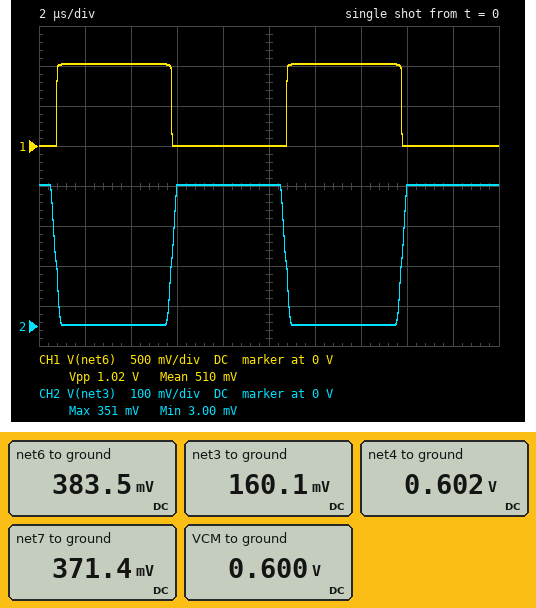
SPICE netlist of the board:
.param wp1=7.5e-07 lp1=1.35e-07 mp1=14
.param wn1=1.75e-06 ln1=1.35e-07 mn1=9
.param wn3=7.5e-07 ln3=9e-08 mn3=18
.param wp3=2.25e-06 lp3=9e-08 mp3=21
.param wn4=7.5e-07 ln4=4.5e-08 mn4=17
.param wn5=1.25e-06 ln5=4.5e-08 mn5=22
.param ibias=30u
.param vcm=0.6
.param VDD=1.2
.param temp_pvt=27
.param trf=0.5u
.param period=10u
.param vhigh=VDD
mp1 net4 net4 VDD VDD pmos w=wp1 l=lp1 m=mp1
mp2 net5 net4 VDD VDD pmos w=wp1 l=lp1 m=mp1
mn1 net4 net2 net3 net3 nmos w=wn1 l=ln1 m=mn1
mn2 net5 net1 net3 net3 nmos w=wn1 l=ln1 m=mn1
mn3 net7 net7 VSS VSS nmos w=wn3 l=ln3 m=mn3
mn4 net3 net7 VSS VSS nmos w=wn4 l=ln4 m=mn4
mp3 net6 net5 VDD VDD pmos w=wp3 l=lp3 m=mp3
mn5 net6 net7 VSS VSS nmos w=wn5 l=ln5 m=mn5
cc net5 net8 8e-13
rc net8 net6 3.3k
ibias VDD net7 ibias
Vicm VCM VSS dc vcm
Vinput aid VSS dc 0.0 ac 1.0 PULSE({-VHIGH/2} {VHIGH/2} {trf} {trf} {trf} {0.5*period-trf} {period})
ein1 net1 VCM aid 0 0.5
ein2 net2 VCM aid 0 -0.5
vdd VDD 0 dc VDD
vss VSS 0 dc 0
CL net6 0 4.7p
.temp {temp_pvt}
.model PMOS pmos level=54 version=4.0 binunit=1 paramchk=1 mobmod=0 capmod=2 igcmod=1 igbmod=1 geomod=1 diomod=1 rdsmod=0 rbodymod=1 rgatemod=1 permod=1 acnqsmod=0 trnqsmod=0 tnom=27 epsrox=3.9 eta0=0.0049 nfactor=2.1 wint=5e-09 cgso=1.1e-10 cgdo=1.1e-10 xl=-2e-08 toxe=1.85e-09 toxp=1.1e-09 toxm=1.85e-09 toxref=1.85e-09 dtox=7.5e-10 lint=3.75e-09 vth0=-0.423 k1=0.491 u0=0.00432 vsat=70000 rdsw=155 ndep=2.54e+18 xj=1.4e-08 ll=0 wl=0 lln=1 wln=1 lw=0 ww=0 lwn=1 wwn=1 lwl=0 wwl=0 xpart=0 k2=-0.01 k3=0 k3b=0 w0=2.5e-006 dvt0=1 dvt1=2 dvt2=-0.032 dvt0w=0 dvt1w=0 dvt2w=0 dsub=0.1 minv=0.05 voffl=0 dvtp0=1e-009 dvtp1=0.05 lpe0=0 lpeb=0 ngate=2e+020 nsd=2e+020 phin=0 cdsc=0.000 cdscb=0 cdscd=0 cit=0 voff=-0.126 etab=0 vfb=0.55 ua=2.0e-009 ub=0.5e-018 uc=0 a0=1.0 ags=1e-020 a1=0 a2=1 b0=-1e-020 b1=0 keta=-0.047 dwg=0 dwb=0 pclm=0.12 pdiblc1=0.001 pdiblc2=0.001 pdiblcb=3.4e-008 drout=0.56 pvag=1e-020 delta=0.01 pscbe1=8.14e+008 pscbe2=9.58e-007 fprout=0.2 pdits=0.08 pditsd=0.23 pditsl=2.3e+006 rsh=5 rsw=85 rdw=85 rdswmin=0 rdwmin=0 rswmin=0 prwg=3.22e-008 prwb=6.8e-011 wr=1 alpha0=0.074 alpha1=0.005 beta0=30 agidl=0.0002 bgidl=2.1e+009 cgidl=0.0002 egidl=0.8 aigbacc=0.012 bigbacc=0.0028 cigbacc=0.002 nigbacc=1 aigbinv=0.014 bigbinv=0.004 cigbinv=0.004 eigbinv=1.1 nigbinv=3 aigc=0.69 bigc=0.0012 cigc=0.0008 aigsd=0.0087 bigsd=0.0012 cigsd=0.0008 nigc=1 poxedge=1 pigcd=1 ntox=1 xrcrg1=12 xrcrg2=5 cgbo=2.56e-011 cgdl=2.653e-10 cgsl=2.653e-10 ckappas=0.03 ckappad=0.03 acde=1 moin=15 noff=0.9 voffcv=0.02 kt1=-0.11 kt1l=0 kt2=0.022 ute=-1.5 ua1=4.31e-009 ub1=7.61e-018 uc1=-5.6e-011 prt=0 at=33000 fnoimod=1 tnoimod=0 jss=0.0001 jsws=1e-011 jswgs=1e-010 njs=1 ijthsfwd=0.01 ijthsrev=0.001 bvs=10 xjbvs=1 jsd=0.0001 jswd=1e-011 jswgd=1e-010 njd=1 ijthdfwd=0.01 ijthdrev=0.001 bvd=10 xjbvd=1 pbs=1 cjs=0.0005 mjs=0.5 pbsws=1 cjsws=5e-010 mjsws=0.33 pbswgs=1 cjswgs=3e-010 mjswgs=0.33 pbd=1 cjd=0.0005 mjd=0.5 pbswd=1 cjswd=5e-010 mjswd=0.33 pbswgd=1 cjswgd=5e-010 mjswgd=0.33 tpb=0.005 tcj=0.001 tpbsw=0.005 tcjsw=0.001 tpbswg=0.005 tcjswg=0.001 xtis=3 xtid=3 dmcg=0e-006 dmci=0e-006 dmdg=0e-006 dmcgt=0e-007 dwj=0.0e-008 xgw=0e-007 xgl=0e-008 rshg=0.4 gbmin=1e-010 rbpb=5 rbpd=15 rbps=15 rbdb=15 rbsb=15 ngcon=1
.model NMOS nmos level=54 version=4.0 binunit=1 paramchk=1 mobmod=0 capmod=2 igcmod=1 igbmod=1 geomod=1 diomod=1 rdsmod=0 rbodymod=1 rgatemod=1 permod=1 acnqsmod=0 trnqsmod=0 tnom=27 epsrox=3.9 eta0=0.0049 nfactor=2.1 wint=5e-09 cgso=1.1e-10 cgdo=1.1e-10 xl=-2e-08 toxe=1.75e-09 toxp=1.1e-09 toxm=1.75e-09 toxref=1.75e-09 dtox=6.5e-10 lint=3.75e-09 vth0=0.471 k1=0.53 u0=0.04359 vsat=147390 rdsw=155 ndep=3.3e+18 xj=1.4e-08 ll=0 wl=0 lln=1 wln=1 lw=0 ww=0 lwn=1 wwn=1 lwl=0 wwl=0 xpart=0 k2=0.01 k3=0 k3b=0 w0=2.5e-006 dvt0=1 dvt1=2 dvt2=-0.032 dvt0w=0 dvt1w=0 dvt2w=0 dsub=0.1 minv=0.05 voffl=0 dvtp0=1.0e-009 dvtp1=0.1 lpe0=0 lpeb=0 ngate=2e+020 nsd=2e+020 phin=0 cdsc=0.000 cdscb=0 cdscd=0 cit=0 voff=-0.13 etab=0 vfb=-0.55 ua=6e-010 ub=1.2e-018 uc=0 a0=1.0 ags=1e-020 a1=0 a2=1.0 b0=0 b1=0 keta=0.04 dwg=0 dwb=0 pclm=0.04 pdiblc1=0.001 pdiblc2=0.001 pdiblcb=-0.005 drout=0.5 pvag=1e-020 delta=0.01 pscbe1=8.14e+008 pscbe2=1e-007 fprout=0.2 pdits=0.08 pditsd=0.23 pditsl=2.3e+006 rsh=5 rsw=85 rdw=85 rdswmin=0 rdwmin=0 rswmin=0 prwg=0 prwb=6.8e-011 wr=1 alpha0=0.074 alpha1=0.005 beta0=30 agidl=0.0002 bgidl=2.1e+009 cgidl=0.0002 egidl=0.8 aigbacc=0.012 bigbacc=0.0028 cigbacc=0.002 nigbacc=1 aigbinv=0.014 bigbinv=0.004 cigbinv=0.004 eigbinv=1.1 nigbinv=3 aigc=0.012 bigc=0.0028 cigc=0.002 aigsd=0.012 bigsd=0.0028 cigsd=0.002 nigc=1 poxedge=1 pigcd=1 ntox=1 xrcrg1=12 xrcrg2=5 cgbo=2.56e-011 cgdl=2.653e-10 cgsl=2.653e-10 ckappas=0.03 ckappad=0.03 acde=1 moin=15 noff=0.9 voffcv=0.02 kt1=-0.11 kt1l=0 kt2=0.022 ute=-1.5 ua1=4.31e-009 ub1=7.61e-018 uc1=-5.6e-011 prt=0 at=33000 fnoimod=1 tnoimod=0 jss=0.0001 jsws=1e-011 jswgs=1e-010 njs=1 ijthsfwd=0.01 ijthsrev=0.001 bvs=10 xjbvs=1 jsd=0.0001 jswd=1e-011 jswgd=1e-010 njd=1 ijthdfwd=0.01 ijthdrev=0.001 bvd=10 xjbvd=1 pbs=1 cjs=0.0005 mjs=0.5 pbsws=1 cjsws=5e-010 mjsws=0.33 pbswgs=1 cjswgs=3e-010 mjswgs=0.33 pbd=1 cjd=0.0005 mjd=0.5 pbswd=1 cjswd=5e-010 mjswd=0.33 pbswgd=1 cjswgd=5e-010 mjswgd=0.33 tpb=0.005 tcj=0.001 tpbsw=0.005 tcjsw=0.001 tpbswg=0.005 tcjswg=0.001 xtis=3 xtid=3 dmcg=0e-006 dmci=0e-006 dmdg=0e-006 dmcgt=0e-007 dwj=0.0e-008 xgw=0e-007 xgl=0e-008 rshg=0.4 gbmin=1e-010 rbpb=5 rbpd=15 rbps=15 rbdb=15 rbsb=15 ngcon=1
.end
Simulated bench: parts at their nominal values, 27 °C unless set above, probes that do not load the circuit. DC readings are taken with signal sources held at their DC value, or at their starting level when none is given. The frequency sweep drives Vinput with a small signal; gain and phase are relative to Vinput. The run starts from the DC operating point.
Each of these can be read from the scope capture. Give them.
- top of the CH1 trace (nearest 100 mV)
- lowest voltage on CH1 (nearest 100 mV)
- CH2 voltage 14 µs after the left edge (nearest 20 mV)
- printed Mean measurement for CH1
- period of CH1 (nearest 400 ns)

1.0 V
0 V
0 V
510 mV
10.0 µs
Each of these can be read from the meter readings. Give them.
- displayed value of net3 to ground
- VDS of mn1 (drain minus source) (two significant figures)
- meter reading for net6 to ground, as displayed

160.1 mV
440 mV
383.5 mV
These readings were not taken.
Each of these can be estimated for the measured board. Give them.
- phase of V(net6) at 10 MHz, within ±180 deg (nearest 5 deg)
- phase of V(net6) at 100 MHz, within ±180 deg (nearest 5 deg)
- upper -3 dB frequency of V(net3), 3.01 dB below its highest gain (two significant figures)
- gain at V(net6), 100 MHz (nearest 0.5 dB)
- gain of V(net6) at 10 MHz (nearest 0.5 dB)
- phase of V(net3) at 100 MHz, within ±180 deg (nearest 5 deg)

-80 deg
-65 deg
910 kHz
10.0 dB
25.5 dB
-160 deg
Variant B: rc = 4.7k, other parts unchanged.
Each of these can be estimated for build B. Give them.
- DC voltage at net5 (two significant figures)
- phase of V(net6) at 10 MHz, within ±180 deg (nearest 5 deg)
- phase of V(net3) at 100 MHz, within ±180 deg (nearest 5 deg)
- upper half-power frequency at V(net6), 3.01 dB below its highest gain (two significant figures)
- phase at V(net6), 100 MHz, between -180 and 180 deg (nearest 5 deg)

600 mV
-75 deg
-155 deg
900 kHz
-60 deg
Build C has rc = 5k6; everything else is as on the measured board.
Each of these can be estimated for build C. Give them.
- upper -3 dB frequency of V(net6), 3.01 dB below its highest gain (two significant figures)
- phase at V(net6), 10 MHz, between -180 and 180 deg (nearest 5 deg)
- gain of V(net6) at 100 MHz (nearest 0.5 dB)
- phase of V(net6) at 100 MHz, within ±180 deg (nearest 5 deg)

900 kHz
-75 deg
14.0 dB
-55 deg
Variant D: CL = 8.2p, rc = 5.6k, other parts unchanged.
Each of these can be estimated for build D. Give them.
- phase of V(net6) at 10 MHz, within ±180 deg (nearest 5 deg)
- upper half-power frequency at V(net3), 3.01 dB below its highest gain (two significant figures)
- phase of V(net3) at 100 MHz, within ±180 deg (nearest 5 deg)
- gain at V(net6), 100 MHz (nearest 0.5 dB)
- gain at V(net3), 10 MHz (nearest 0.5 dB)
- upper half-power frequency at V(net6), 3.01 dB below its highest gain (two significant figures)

-75 deg
900 kHz
-165 deg
13.0 dB
-30.5 dB
890 kHz
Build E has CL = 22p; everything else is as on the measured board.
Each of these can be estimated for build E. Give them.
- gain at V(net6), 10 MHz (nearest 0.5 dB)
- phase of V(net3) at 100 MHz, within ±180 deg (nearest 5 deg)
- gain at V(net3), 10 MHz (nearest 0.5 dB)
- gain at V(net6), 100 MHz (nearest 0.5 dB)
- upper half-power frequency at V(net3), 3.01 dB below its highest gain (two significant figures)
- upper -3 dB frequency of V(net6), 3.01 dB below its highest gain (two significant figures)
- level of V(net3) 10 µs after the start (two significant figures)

25.0 dB
165 deg
-29.0 dB
4.0 dB
890 kHz
880 kHz
350 mV
